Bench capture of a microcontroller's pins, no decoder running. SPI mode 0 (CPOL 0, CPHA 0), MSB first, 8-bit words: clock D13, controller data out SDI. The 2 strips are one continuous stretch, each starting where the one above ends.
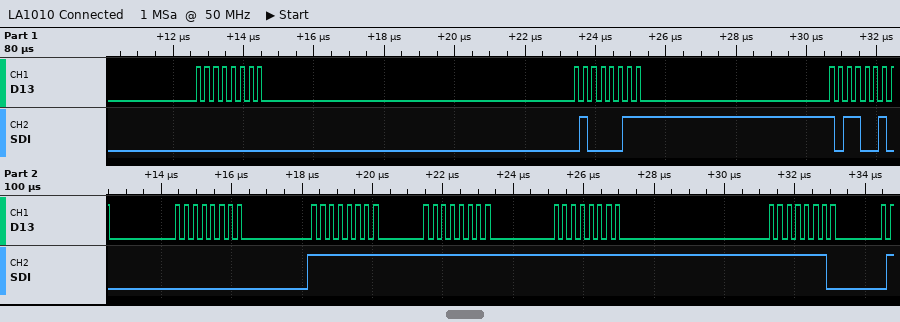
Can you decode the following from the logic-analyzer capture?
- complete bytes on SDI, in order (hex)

00 43 B2 00 FF FF FF FE
